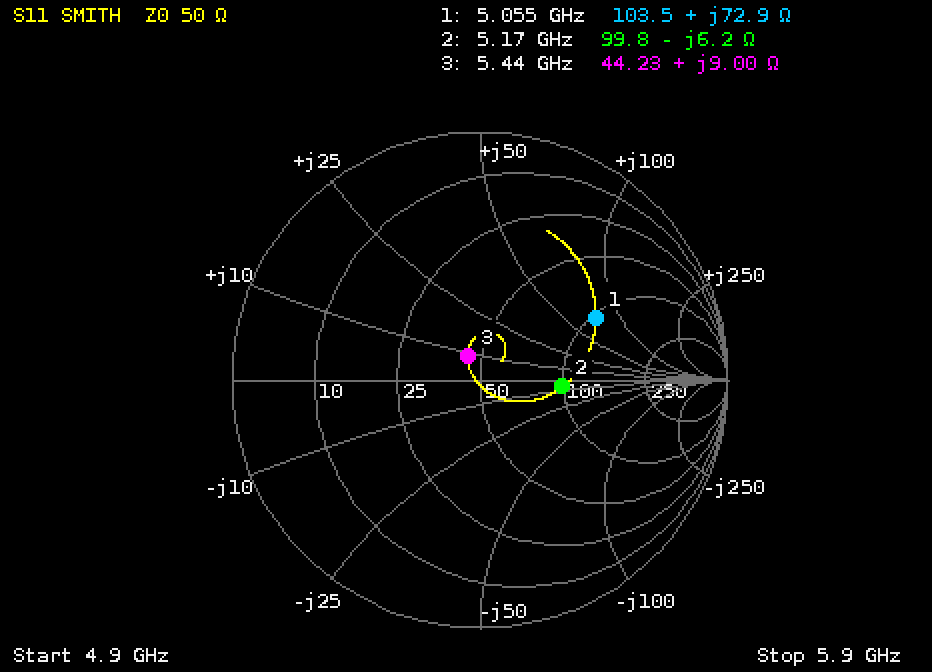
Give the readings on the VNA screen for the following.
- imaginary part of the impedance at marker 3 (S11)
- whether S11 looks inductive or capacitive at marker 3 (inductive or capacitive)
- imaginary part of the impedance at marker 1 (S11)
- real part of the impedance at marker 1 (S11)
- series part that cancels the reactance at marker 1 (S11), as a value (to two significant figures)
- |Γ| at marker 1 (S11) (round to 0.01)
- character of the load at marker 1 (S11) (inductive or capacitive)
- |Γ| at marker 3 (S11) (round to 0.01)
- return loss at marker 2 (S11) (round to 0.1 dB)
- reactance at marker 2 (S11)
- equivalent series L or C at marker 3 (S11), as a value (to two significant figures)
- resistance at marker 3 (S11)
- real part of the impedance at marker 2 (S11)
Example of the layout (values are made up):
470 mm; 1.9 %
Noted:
+9.00 Ω; inductive; +72.9 Ω; 103.5 Ω; 430 fF; 0.53; inductive; 0.11; 9.5 dB; -6.2 Ω; 260 pH; 44.23 Ω; 99.8 Ω
